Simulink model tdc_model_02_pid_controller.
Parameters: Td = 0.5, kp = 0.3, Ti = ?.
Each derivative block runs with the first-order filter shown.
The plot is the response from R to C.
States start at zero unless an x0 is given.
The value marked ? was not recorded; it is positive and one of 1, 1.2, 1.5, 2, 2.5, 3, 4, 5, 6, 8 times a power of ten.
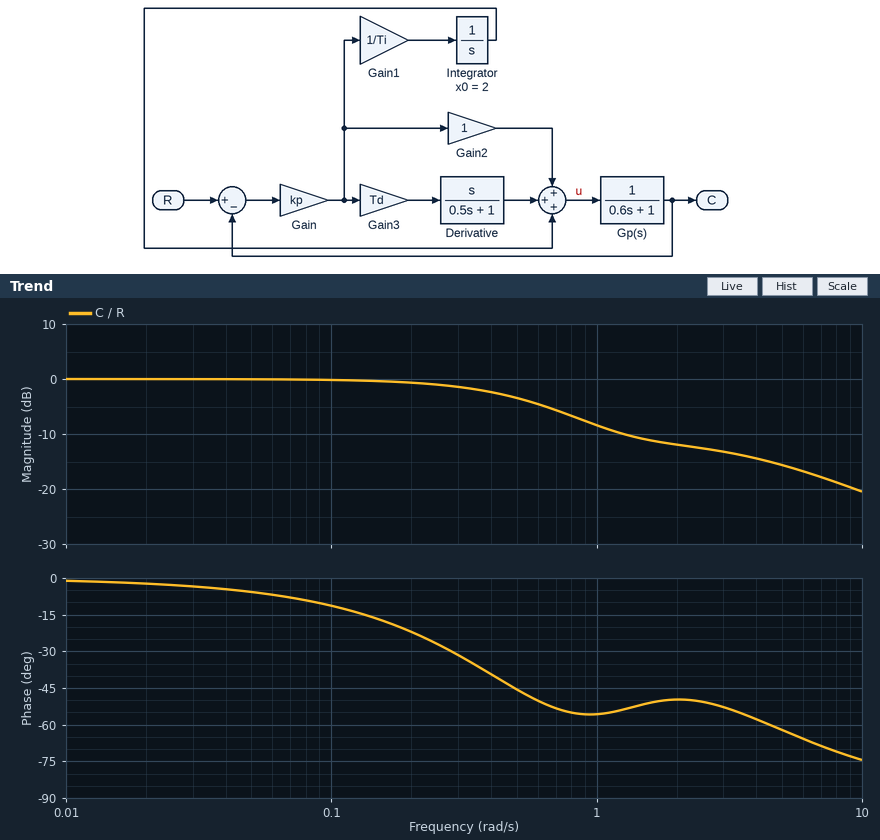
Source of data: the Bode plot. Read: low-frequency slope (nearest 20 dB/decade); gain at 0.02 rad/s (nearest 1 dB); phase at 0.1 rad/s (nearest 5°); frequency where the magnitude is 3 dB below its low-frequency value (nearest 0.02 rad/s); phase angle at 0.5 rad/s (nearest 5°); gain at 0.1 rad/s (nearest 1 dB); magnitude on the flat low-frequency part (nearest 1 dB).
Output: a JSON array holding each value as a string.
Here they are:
["0 dB/decade", "0 dB", "-10°", "0.46 rad/s", "-45°", "0 dB", "0 dB"]
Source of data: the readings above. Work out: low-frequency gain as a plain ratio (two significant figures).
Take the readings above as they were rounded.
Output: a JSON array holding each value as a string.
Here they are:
["1.0"]
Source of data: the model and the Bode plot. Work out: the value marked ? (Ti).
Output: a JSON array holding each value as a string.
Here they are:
["0.6"]
